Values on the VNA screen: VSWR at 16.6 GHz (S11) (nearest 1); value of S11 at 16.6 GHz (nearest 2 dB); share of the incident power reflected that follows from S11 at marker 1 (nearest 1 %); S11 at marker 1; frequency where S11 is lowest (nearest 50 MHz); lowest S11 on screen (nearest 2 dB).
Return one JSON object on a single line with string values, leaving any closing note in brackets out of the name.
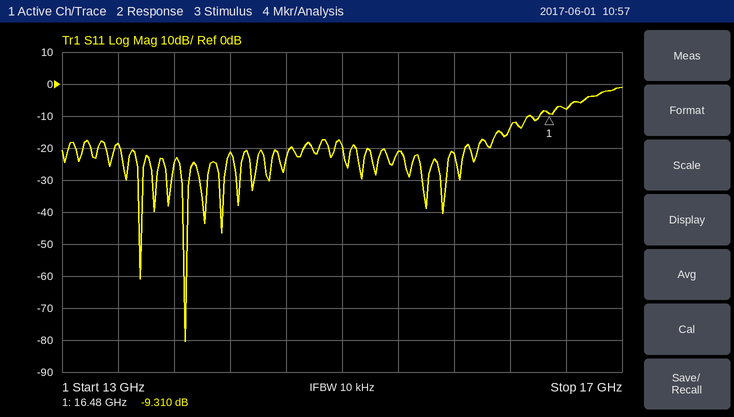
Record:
{"VSWR at 16.6 GHz (S11)": "2", "value of S11 at 16.6 GHz": "-8 dB", "share of the incident power reflected that follows from S11 at marker 1": "12 %", "S11 at marker 1": "-9.310 dB", "frequency where S11 is lowest": "13.90 GHz", "lowest S11 on screen": "-80 dB"}
